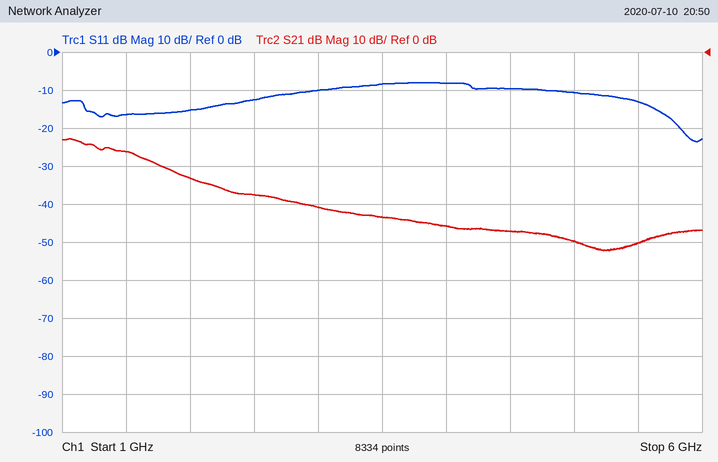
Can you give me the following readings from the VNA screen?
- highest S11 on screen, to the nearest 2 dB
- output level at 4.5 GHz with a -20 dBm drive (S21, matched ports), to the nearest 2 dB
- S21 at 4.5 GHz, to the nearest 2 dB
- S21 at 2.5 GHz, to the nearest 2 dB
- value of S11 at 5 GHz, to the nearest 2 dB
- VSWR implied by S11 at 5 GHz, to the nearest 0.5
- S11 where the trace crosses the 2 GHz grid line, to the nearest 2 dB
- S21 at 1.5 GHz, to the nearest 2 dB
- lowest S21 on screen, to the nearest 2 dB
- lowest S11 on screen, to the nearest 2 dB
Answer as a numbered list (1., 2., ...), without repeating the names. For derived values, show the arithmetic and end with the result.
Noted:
1. -8 dB
2. -20 dBm + (-48 dB) = -68 dBm
3. -48 dB
4. -38 dB
5. -10 dB
6. |Γ| = 10^(-10/20) = 0.3162; VSWR = (1 + 0.3162)/(1 − 0.3162) ≈ 1.92, so 2.0 to the nearest 0.5
7. -16 dB
8. -26 dB
9. -52 dB
10. -24 dB
